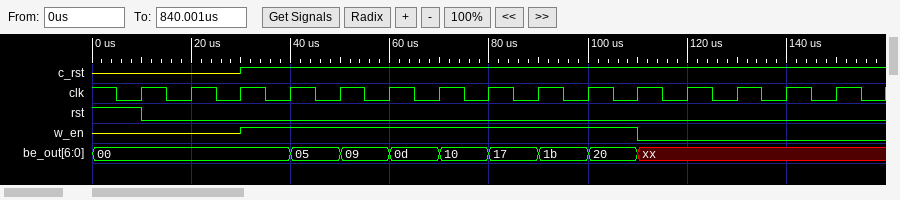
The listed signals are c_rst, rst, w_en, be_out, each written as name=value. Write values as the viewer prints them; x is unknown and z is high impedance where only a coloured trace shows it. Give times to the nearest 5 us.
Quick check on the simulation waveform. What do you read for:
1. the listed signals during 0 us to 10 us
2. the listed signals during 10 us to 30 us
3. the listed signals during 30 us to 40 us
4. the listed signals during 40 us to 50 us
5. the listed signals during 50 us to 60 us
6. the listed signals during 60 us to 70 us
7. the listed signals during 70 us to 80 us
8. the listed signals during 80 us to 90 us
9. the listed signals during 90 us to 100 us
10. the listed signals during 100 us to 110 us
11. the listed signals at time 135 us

c_rst=z, rst=1, w_en=z, be_out=00
c_rst=z, rst=0, w_en=z, be_out=00
c_rst=1, rst=0, w_en=1, be_out=00
c_rst=1, rst=0, w_en=1, be_out=05
c_rst=1, rst=0, w_en=1, be_out=09
c_rst=1, rst=0, w_en=1, be_out=0d
c_rst=1, rst=0, w_en=1, be_out=10
c_rst=1, rst=0, w_en=1, be_out=17
c_rst=1, rst=0, w_en=1, be_out=1b
c_rst=1, rst=0, w_en=1, be_out=20
c_rst=1, rst=0, w_en=0, be_out=xx
